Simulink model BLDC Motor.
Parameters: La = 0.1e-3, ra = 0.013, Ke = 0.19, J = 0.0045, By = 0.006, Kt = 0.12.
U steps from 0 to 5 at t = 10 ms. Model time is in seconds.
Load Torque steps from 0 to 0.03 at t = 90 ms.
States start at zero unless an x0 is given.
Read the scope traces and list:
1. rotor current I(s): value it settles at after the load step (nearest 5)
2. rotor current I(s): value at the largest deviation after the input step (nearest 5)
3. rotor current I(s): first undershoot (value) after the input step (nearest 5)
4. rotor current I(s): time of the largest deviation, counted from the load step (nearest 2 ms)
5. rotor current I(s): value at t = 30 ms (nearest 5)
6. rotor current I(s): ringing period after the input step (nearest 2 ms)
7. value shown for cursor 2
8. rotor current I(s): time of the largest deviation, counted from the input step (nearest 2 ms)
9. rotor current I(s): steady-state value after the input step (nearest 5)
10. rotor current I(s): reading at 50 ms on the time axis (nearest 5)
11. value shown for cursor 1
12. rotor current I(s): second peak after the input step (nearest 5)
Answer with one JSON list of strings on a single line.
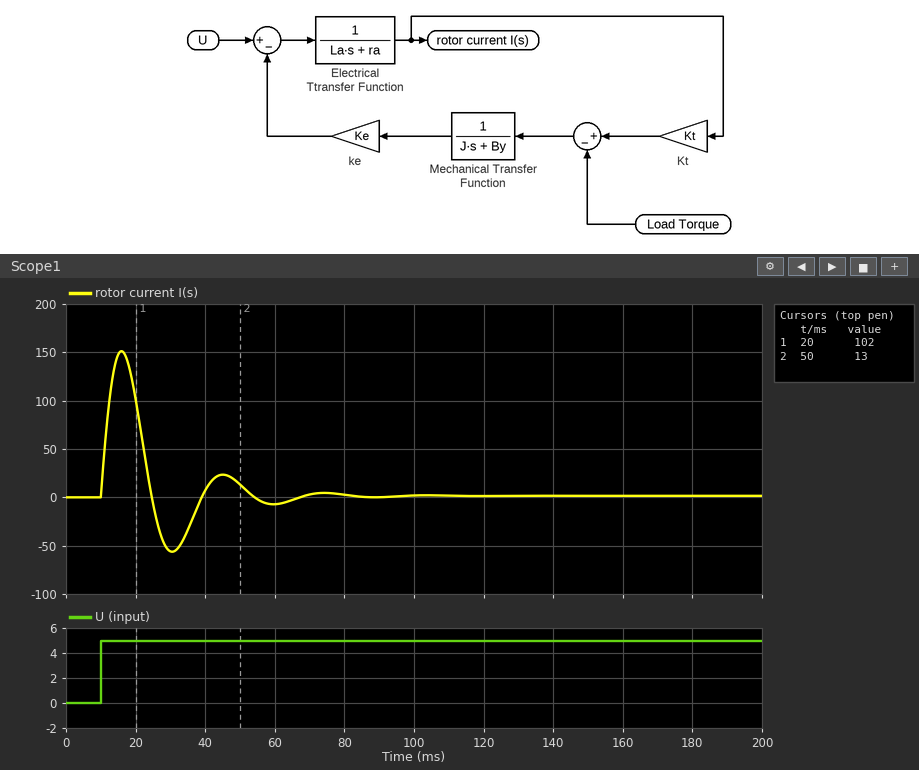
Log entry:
["0", "150", "-55", "14 ms", "-55", "30 ms", "13", "6 ms", "0", "15", "102", "25"]
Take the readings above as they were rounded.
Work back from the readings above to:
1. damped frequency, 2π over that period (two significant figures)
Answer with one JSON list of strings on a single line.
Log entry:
["0.21 rad/ms"]
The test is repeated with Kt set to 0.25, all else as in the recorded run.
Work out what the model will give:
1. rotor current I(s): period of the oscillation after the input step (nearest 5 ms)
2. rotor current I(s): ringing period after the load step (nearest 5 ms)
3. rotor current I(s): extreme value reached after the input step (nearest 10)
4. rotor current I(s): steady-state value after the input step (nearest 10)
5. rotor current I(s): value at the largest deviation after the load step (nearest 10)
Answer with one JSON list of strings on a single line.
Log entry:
["20 ms", "20 ms", "120", "0", "0"]
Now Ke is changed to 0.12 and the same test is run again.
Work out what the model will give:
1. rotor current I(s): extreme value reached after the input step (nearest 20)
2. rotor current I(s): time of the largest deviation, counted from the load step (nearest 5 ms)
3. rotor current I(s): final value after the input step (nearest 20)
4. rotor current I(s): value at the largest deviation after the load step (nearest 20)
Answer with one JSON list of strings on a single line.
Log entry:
["180", "20 ms", "0", "0"]
